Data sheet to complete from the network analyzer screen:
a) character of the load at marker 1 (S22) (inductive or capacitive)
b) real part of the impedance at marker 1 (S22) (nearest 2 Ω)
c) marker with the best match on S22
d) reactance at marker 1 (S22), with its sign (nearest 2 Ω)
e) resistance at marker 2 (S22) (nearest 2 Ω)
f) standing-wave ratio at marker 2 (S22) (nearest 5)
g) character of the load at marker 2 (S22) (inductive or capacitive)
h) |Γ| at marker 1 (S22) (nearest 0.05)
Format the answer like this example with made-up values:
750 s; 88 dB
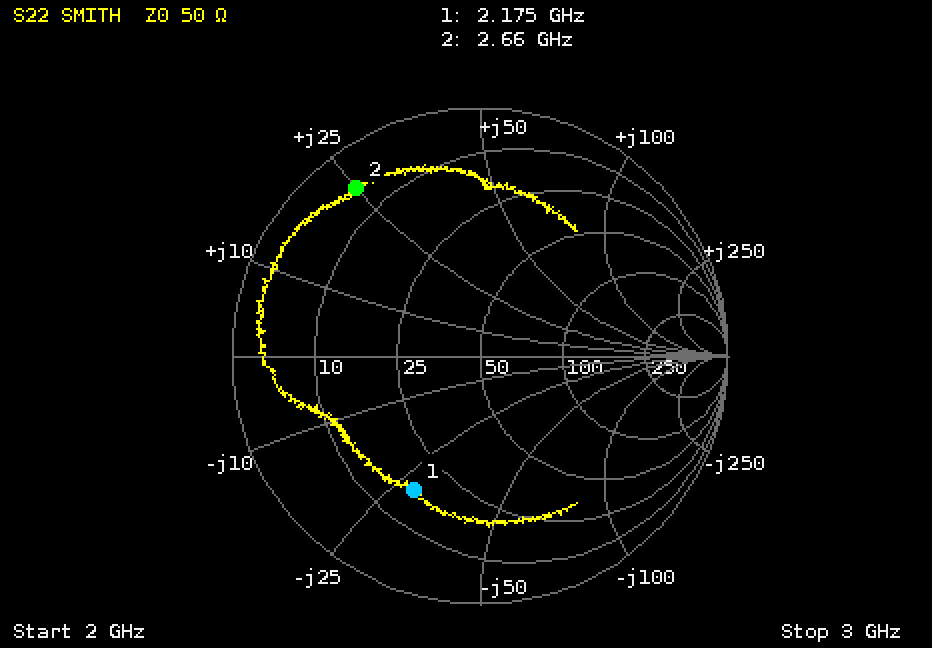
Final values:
capacitive; 16 Ω; marker 1; -28 Ω; 6 Ω; 10; inductive; 0.60
